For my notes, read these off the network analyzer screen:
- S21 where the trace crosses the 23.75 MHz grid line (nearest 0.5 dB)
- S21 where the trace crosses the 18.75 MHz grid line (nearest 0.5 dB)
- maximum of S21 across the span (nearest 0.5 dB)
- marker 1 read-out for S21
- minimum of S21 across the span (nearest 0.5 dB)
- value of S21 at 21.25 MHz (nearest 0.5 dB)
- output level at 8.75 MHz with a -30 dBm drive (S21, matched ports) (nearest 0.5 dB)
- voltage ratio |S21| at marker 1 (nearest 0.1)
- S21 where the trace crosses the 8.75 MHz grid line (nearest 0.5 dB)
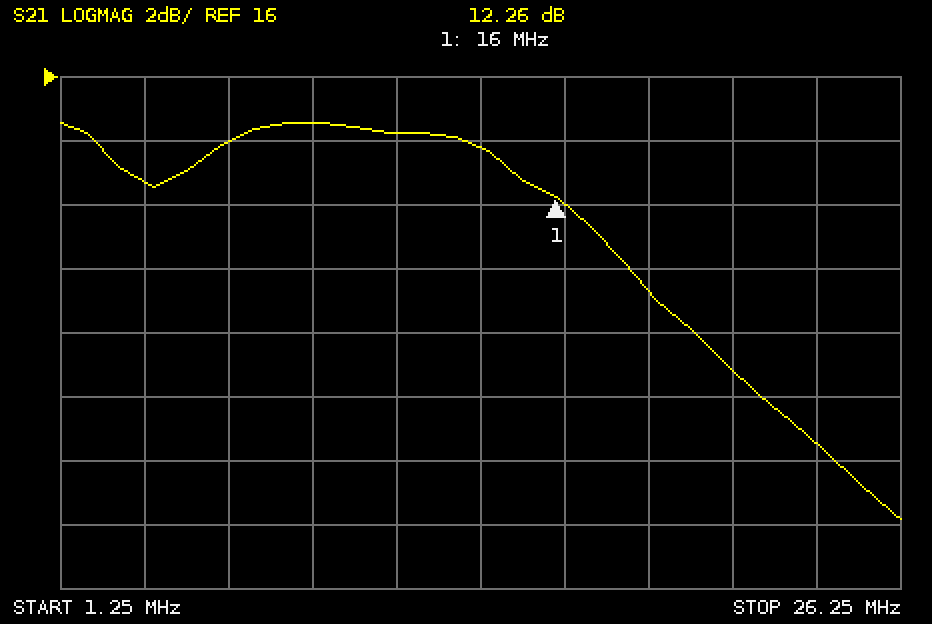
4.5 dB
9.5 dB
14.5 dB
12.26 dB
2.0 dB
7.0 dB
-15.5 dBm
4.1
14.5 dB
